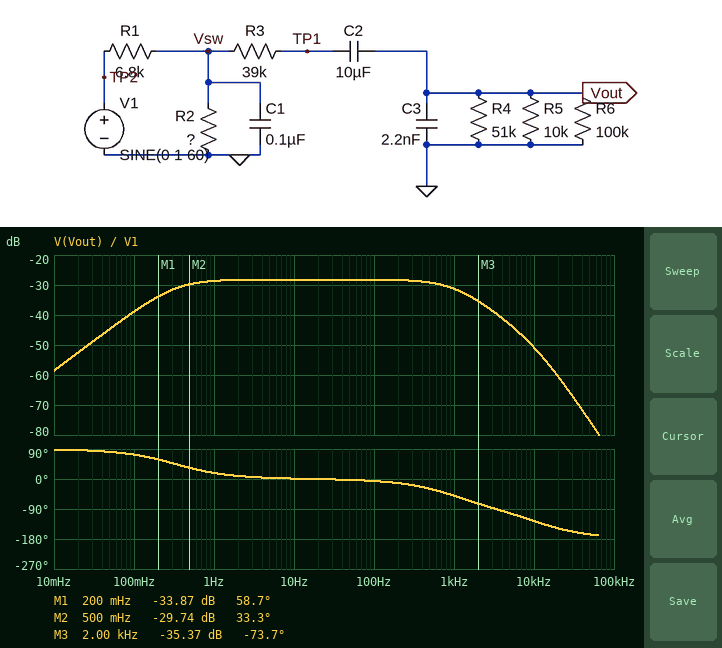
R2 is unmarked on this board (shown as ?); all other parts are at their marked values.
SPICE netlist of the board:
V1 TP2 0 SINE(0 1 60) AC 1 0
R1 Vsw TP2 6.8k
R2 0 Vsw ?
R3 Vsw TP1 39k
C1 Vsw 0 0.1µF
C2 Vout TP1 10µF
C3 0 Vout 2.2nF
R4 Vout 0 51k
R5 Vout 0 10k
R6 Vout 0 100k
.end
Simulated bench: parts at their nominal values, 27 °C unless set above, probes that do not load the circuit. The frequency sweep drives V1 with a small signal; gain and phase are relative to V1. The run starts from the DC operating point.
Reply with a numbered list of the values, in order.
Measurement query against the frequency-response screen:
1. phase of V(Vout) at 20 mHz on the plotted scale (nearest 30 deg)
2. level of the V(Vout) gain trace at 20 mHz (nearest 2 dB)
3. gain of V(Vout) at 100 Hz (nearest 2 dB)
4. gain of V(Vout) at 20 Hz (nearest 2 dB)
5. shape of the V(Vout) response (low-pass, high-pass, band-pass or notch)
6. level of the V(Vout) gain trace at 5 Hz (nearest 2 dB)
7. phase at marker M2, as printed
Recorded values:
1. 90 deg
2. -52 dB
3. -28 dB
4. -28 dB
5. band-pass
6. -28 dB
7. 33.3 deg
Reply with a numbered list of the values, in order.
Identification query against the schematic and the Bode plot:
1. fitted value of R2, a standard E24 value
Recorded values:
1. 2.2 kΩ
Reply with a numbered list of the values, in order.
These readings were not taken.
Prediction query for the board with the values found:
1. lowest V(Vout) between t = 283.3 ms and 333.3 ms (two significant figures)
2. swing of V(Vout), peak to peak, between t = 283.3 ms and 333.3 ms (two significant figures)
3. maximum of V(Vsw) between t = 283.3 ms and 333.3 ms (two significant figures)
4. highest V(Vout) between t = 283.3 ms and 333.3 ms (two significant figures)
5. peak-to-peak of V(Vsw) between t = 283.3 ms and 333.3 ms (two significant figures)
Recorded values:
1. -39 mV
2. 78 mV
3. 240 mV
4. 39 mV
5. 470 mV
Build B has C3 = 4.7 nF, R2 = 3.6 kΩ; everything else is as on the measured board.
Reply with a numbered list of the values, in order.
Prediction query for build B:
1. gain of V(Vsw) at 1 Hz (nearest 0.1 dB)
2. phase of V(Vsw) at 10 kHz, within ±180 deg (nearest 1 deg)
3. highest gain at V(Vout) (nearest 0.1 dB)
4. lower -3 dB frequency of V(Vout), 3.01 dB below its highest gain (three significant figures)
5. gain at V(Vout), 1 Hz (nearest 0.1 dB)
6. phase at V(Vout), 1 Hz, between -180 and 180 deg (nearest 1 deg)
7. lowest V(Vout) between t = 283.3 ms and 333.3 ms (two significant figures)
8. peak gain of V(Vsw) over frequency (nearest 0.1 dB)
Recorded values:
1. -9.6 dB
2. -86 deg
3. -25.3 dB
4. 324 mHz
5. -25.7 dB
6. 18 deg
7. -54 mV
8. -9.2 dB
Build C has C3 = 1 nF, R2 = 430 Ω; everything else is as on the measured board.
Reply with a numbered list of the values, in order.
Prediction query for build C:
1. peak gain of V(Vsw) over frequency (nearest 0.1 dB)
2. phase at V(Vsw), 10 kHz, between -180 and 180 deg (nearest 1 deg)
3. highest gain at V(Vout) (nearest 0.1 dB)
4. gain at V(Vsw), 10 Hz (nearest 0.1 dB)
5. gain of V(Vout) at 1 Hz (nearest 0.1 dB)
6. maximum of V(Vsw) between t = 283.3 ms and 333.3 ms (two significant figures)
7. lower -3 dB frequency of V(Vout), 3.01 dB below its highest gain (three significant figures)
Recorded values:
1. -24.5 dB
2. -68 deg
3. -40.2 dB
4. -24.6 dB
5. -40.7 dB
6. 59 mV
7. 338 mHz
